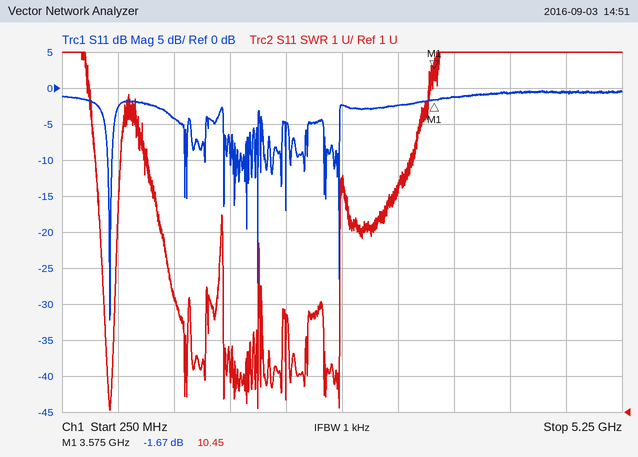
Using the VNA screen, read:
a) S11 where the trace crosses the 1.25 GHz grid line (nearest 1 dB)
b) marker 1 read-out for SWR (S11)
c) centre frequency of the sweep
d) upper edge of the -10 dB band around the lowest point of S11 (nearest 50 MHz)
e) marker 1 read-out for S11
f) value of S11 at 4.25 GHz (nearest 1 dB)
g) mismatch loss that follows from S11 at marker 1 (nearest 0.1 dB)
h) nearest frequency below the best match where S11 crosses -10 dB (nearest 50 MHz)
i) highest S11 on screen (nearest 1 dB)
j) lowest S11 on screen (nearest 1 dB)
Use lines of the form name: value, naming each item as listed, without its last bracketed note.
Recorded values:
S11 where the trace crosses the 1.25 GHz grid line: -4 dB
marker 1 read-out for SWR: 10.45
centre frequency of the sweep: 2.75 GHz
upper edge of the -10 dB band around the lowest point of S11: 700 MHz
marker 1 read-out for S11: -1.67 dB
value of S11 at 4.25 GHz: -1 dB
mismatch loss that follows from S11 at marker 1: 5.0 dB
nearest frequency below the best match where S11 crosses -10 dB: 650 MHz
highest S11 on screen: 0 dB
lowest S11 on screen: -32 dB
